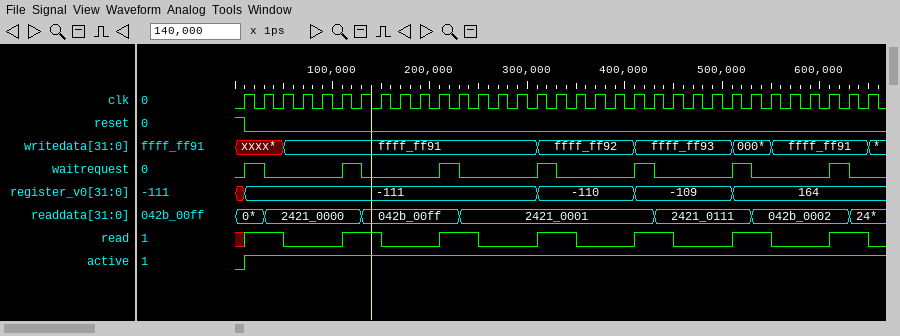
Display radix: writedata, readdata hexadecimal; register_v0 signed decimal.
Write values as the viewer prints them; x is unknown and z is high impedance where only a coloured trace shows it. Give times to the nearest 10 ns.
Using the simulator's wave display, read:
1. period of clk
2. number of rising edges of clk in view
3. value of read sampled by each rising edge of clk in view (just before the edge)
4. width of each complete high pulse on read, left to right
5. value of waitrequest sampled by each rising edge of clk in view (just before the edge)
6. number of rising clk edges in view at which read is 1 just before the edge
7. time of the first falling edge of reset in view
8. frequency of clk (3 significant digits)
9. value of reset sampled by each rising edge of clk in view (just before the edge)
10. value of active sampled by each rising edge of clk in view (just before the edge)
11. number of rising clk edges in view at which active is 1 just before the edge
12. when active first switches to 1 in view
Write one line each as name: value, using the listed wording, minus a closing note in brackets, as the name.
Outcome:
period of clk: 20 ns
number of rising edges of clk in view: 33
value of read sampled by each rising edge of clk in view: x 1 1 0 0 0 1 1 0 0 0 1 1 0 0 0 1 1 0 0 0 1 1 0 0 0 1 1 0 0 0 1 1
width of each complete high pulse on read, left to right: 40 ns, 40 ns, 40 ns, 40 ns, 40 ns, 40 ns
value of waitrequest sampled by each rising edge of clk in view: 0 1 0 0 0 0 1 0 0 0 0 1 0 0 0 0 1 0 0 0 0 1 0 0 0 0 1 0 0 0 0 1 0
number of rising clk edges in view at which read is 1 just before the edge: 14
time of the first falling edge of reset in view: 10 ns
frequency of clk: 50.0 MHz
value of reset sampled by each rising edge of clk in view: 1 0 0 0 0 0 0 0 0 0 0 0 0 0 0 0 0 0 0 0 0 0 0 0 0 0 0 0 0 0 0 0 0
value of active sampled by each rising edge of clk in view: 0 1 1 1 1 1 1 1 1 1 1 1 1 1 1 1 1 1 1 1 1 1 1 1 1 1 1 1 1 1 1 1 1
number of rising clk edges in view at which active is 1 just before the edge: 32
when active first switches to 1 in view: 10 ns
